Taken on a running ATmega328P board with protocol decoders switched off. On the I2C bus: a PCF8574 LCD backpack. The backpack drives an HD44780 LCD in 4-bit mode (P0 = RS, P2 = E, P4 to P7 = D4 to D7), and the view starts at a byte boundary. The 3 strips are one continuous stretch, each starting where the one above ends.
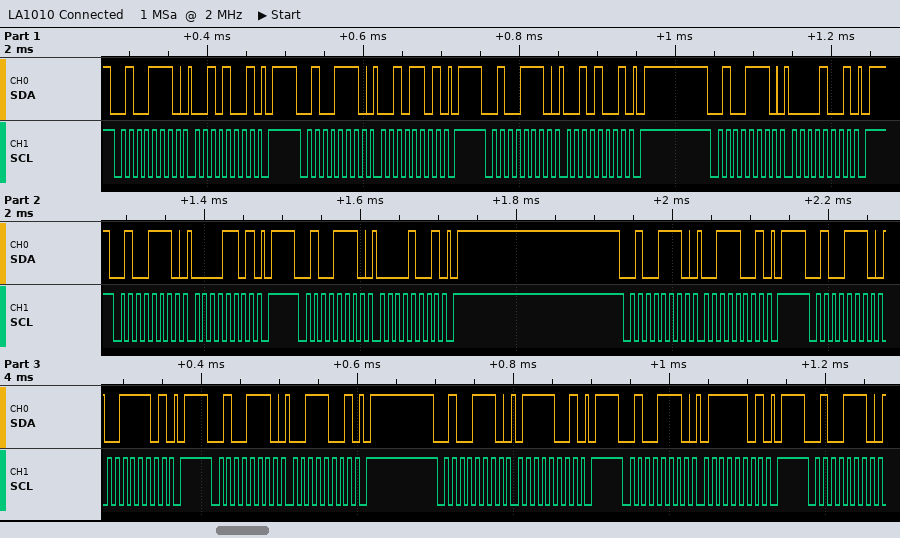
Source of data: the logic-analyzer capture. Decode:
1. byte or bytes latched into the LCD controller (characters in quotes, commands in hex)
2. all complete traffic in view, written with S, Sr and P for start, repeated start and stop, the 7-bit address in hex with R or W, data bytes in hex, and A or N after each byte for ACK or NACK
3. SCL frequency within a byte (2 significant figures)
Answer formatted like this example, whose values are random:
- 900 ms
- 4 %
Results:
- ' '
- S 27W A 29 A P S 27W A 2D A P S 27W A 29 A P S 27W A 09 A P S 27W A 0D A P S 27W A 09 A P S 27W A 39 A P S 27W A 3D A P S 27W A 39 A P S 27W A 79 A P S 27W A 7D A P S 27W A
- 100 kHz
